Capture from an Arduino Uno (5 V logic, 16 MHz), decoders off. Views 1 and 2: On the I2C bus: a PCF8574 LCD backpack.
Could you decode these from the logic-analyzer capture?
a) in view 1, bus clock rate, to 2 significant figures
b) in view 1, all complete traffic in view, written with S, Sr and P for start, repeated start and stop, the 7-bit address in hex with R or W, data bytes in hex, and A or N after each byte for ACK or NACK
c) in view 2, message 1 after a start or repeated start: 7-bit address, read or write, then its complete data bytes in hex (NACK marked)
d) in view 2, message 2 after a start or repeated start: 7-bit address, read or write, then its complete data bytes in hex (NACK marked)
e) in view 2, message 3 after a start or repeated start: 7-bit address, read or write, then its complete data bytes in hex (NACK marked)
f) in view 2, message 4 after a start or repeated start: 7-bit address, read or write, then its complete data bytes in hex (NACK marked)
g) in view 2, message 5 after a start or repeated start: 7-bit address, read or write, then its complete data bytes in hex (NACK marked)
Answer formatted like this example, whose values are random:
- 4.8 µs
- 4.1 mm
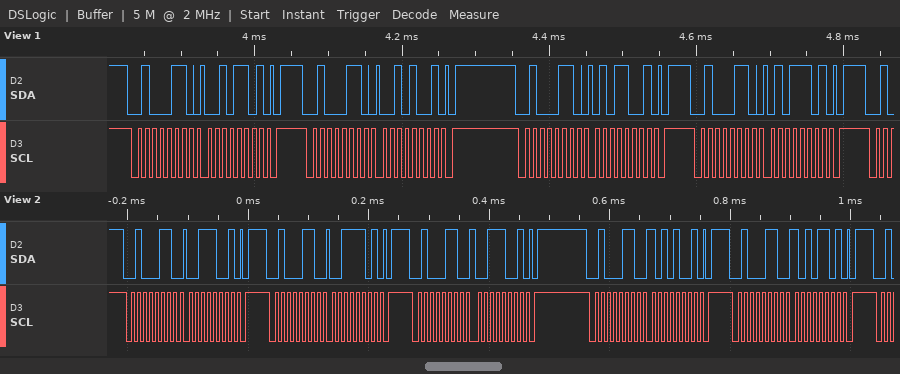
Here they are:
- 100 kHz
- S 23W A 2D A P S 23W A 29 A P S 23W A 59 A P S 23W A 5D A P
- 0x23 write: 39
- 0x23 write: 3D
- 0x23 write: 39
- 0x23 write: A9
- 0x23 write: AD
